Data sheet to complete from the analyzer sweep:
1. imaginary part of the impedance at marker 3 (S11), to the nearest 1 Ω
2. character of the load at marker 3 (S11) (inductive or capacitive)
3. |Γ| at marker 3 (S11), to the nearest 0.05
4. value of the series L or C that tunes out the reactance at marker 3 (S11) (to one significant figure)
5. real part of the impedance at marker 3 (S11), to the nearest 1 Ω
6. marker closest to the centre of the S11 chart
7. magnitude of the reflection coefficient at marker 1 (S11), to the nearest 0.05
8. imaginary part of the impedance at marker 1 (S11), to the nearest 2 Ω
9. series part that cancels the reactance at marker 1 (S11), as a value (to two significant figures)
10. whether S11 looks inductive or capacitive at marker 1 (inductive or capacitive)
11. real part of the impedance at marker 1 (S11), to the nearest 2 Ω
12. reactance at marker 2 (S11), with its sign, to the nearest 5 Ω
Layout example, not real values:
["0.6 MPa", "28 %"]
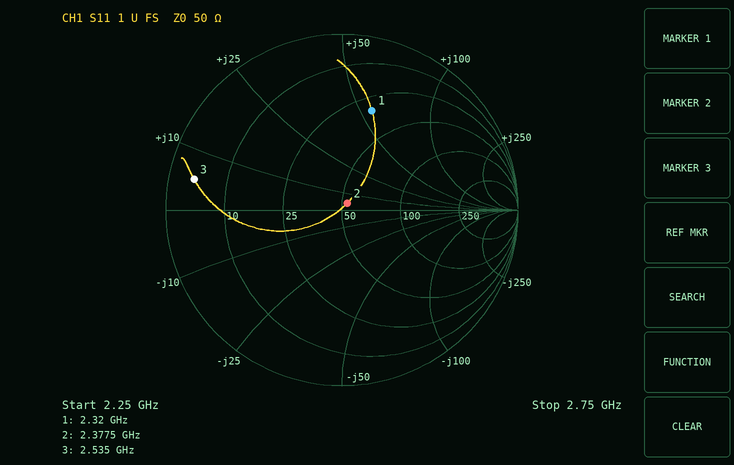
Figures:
["+5 Ω", "inductive", "0.85", "10 pF", "4 Ω", "marker 2", "0.60", "+56 Ω", "1.2 pF", "inductive", "32 Ω", "+5 Ω"]
